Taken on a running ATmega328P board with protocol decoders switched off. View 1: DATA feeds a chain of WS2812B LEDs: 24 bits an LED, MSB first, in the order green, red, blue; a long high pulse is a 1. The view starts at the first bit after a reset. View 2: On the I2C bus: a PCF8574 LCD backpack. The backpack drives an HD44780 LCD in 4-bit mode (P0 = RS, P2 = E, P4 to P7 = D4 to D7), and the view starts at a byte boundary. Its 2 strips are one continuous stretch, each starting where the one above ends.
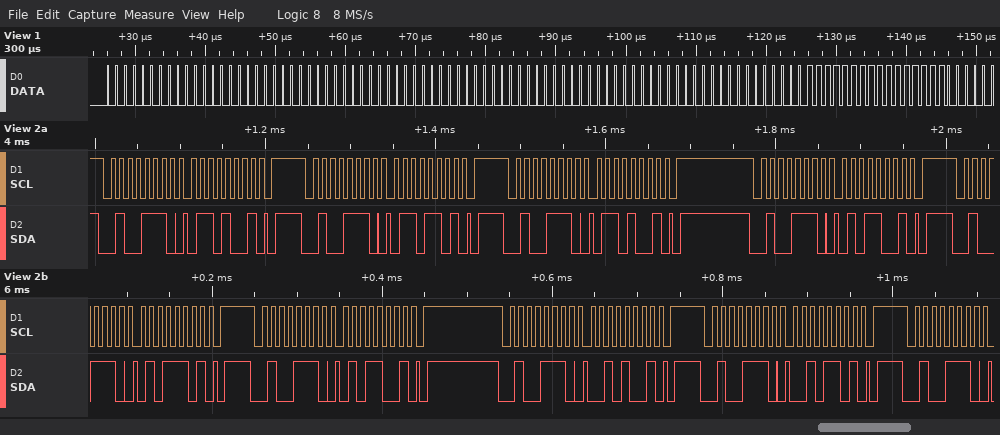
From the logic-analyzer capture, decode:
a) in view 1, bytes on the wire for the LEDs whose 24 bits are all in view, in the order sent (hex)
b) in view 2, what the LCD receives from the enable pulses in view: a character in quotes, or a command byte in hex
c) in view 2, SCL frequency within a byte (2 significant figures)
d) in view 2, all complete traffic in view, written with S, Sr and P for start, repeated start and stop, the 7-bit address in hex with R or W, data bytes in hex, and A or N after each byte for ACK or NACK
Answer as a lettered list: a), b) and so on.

a) 00 00 00 00 00 00 00 00 00 00 FF FF
b) 'e'
c) 100 kHz
d) S 27W A 69 A P S 27W A 6D A P S 27W A 69 A P S 27W A 59 A P S 27W A 5D A P S 27W A 59 A P S 27W A 29 A P S 27W A 2D A P S 27W A
